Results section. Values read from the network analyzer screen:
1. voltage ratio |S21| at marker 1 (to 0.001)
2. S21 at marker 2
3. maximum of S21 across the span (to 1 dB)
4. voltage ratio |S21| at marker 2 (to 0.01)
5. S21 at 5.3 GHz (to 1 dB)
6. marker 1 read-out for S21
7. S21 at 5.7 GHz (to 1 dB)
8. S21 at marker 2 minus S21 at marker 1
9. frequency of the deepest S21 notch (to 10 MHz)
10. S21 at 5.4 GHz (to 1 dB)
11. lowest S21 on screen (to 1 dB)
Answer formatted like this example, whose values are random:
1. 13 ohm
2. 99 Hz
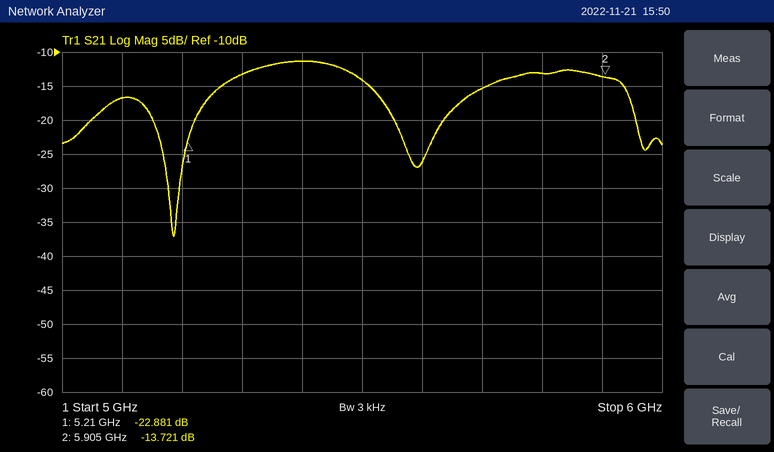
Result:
1. 0.072
2. -13.721 dB
3. -11 dB
4. 0.21
5. -13 dB
6. -22.881 dB
7. -15 dB
8. 9.160 dB
9. 5.19 GHz
10. -11 dB
11. -37 dB
